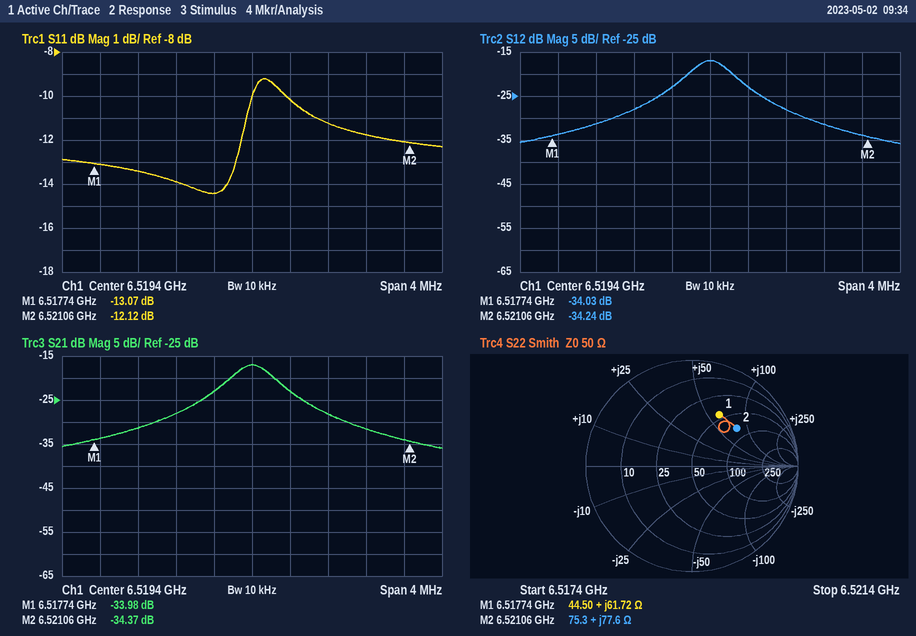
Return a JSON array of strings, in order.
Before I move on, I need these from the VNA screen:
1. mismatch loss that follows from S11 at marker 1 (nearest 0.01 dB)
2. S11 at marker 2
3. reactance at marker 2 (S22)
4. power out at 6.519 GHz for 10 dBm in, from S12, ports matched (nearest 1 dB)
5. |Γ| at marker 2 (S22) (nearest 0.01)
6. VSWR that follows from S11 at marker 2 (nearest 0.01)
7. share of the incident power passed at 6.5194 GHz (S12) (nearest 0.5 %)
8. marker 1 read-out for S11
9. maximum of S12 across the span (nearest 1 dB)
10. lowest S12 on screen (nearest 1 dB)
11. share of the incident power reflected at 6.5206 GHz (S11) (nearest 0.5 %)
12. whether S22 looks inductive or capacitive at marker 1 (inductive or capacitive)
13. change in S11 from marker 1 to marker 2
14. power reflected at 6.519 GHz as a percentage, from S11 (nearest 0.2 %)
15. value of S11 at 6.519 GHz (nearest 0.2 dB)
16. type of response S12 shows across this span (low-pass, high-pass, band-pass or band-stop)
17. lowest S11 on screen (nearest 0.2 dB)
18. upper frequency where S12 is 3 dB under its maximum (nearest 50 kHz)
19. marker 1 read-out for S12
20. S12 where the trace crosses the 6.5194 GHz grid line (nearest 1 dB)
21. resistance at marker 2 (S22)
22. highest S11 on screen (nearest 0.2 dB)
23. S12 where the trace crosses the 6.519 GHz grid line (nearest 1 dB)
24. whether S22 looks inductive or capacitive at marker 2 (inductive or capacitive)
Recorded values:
["0.22 dB", "-12.12 dB", "+77.6 Ω", "-13 dBm", "0.55", "1.66", "2.0 %", "-13.07 dB", "-17 dB", "-36 dB", "6.5 %", "inductive", "0.95 dB", "3.6 %", "-14.4 dB", "band-pass", "-14.4 dB", "6.51965 GHz", "-34.03 dB", "-17 dB", "75.3 Ω", "-9.2 dB", "-23 dB", "inductive"]
